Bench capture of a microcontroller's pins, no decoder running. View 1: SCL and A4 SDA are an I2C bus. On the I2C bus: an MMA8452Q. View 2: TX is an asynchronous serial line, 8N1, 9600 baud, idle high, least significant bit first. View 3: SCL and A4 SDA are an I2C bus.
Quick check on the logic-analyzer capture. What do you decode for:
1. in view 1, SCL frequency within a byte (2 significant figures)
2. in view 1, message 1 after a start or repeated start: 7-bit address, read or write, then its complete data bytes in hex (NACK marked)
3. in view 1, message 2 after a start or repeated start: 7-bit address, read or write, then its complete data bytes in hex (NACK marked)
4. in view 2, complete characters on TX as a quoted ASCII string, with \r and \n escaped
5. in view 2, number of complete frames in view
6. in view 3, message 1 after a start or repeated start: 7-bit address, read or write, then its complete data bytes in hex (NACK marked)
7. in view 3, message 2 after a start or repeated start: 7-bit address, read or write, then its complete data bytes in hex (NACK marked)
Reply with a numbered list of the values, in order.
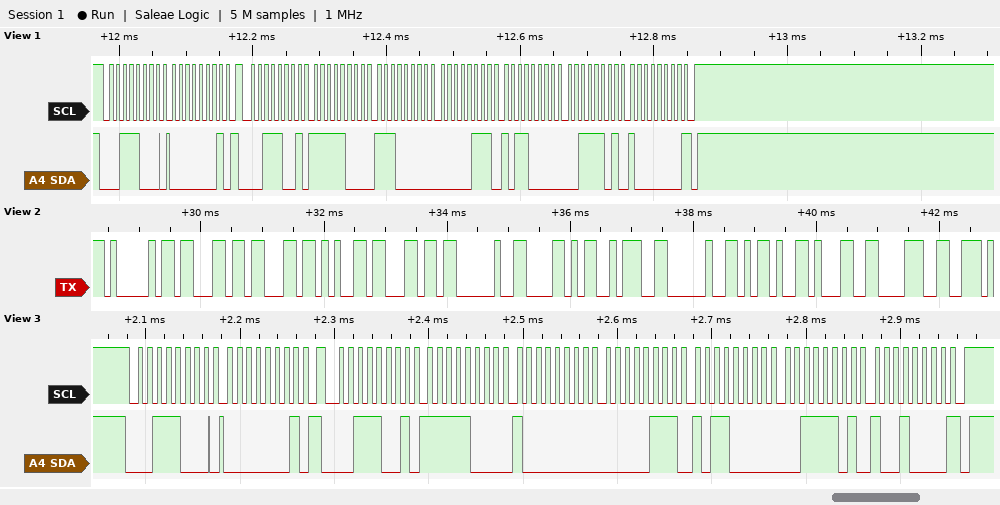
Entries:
1. 100 kHz
2. 0x1C write: 01
3. 0x1C read: F8 E0 07 B0 3D 80 NACK
4. "Accel X: -18"
5. 12
6. 0x1C write: 01
7. 0x1C read: F8 80 07 B0 3D 90 NACK
